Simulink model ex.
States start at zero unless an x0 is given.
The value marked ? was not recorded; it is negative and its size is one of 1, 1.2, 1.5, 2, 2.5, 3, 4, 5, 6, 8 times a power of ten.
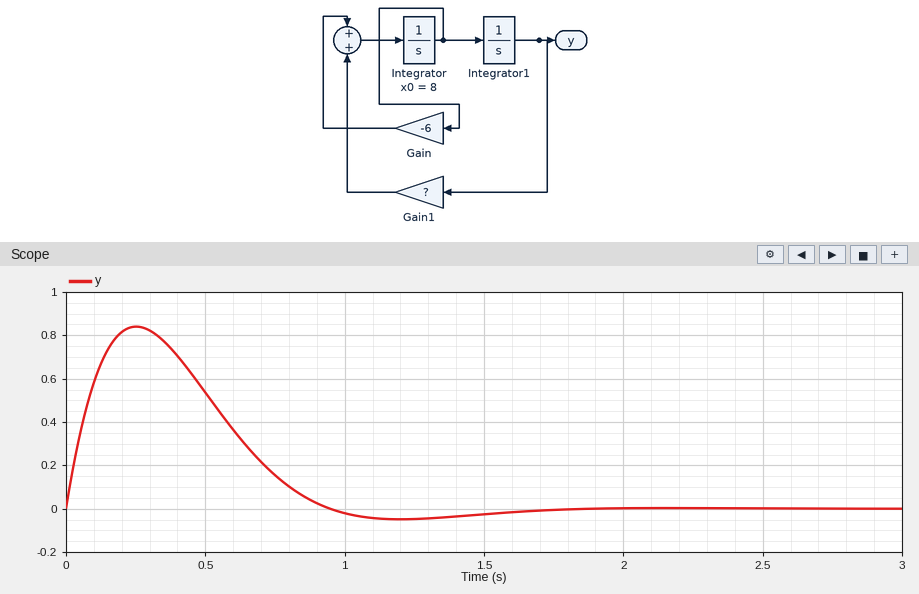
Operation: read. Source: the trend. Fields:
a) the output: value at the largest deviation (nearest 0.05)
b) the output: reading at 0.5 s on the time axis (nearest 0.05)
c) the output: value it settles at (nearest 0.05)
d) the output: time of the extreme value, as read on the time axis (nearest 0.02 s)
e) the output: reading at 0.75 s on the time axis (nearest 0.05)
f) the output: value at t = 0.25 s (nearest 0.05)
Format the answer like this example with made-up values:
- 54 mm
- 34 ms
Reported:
- 0.85
- 0.55
- 0.00
- 0.26 s
- 0.15
- 0.85
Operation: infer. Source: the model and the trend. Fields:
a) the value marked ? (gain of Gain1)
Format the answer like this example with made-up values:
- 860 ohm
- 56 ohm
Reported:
- -20
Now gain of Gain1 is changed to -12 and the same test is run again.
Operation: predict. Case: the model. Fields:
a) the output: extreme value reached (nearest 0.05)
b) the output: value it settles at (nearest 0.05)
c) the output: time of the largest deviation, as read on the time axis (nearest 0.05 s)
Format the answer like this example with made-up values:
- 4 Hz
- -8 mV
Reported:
- 0.95
- 0.00
- 0.30 s
